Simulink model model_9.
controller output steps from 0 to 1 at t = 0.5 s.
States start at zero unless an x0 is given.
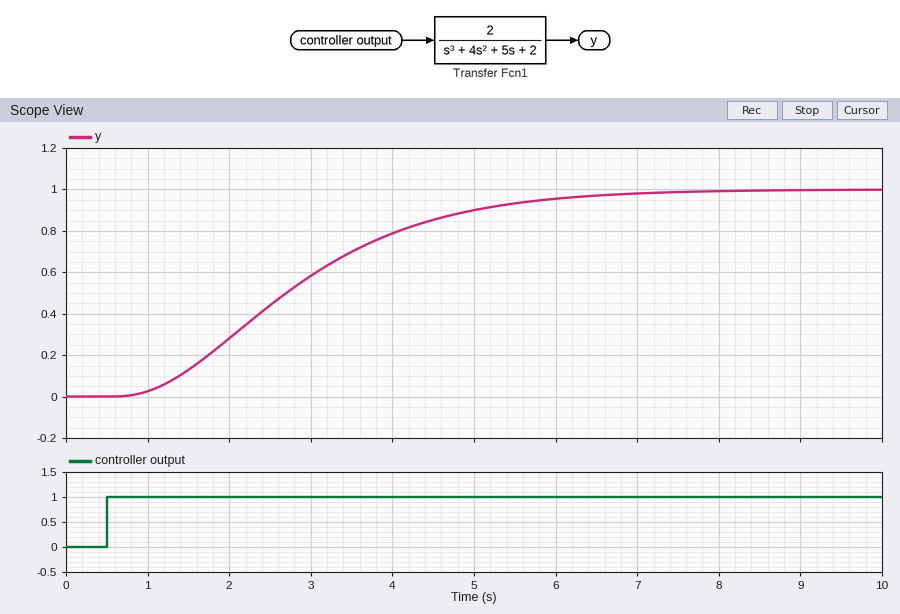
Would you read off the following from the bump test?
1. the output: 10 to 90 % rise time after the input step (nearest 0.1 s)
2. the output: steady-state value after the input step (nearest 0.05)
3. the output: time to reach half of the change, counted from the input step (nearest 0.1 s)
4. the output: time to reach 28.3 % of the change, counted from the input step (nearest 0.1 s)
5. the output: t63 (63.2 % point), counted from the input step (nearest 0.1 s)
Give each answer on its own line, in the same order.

3.6 s
1.00
2.2 s
1.5 s
2.7 s
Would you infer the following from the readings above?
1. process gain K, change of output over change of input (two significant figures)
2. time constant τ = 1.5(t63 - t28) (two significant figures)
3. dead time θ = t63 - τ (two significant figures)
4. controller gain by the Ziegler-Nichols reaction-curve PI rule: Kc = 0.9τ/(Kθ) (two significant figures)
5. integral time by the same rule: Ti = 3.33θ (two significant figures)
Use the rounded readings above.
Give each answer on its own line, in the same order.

1.0
1.8 s
0.90 s
1.8
3.0 s
